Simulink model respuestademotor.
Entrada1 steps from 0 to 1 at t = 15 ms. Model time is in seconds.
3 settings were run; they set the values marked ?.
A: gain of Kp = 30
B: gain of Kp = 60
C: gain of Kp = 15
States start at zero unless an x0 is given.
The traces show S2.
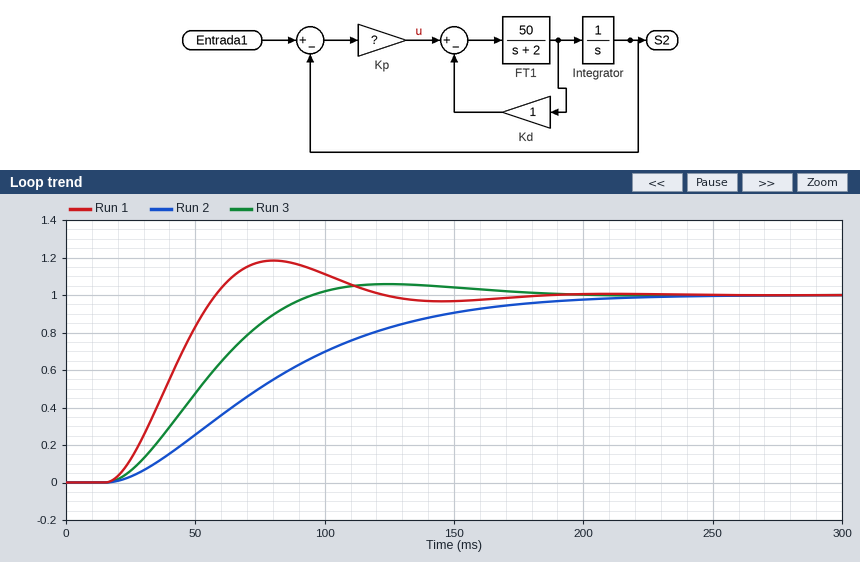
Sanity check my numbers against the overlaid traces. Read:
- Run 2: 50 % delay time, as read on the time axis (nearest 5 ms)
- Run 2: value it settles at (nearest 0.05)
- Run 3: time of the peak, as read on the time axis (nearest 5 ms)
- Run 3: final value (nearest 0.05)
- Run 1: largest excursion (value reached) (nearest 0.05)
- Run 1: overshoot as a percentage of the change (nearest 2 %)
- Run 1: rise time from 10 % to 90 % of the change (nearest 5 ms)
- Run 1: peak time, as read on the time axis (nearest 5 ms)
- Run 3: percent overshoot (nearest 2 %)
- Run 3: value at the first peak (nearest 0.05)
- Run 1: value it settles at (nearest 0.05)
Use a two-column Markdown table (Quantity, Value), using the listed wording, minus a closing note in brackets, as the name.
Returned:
| Quantity | Value |
|---|---|
| Run 2: 50 % delay time, as read on the time axis | 75 ms |
| Run 2: value it settles at | 1.00 |
| Run 3: time of the peak, as read on the time axis | 125 ms |
| Run 3: final value | 1.00 |
| Run 1: largest excursion (value reached) | 1.20 |
| Run 1: overshoot as a percentage of the change | 18 % |
| Run 1: rise time from 10 % to 90 % of the change | 30 ms |
| Run 1: peak time, as read on the time axis | 80 ms |
| Run 3: percent overshoot | 6 % |
| Run 3: value at the first peak | 1.05 |
| Run 1: value it settles at | 1.00 |
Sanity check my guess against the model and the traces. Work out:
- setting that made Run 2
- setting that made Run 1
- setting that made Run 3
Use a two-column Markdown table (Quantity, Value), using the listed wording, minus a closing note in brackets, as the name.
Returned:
| Quantity | Value |
|---|---|
| setting that made Run 2 | C |
| setting that made Run 1 | B |
| setting that made Run 3 | A |
